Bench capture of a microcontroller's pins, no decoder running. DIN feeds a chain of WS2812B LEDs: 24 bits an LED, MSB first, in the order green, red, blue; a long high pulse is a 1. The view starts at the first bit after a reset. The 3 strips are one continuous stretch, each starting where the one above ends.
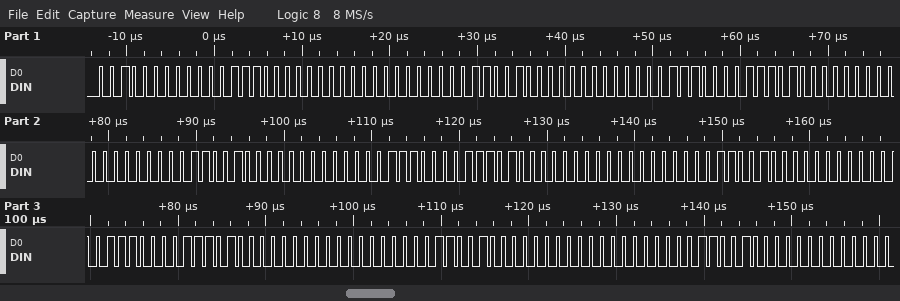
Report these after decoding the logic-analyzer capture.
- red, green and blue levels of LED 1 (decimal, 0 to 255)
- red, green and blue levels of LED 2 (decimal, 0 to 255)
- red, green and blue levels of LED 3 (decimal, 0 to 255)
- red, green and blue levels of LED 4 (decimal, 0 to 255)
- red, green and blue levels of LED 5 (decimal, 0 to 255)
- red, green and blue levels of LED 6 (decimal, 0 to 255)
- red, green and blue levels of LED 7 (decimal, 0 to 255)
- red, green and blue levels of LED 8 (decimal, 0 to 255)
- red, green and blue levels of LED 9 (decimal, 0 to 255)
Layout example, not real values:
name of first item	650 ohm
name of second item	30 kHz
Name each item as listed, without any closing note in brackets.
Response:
red, green and blue levels of LED 1	14, 32, 0
red, green and blue levels of LED 2	50, 0, 0
red, green and blue levels of LED 3	29, 14, 0
red, green and blue levels of LED 4	50, 0, 0
red, green and blue levels of LED 5	29, 14, 0
red, green and blue levels of LED 6	50, 0, 0
red, green and blue levels of LED 7	29, 14, 0
red, green and blue levels of LED 8	50, 0, 0
red, green and blue levels of LED 9	50, 0, 0
